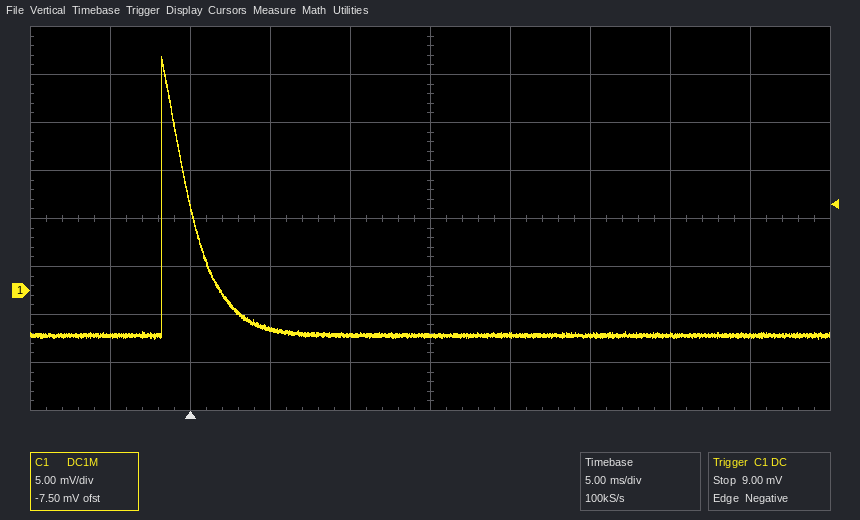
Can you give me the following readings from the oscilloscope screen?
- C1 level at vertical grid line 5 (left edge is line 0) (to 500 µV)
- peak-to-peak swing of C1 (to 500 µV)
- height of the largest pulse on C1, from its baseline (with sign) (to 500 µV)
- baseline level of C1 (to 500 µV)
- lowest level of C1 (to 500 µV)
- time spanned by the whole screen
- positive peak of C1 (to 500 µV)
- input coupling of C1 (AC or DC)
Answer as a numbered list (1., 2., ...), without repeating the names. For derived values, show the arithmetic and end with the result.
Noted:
1. -4.5 mV
2. 24.5 mV − (-5.0 mV) = 29.5 mV
3. 24.5 mV − (-4.5 mV) = +29.0 mV
4. -4.5 mV
5. -5.0 mV
6. 50 ms
7. 24.5 mV
8. DC
